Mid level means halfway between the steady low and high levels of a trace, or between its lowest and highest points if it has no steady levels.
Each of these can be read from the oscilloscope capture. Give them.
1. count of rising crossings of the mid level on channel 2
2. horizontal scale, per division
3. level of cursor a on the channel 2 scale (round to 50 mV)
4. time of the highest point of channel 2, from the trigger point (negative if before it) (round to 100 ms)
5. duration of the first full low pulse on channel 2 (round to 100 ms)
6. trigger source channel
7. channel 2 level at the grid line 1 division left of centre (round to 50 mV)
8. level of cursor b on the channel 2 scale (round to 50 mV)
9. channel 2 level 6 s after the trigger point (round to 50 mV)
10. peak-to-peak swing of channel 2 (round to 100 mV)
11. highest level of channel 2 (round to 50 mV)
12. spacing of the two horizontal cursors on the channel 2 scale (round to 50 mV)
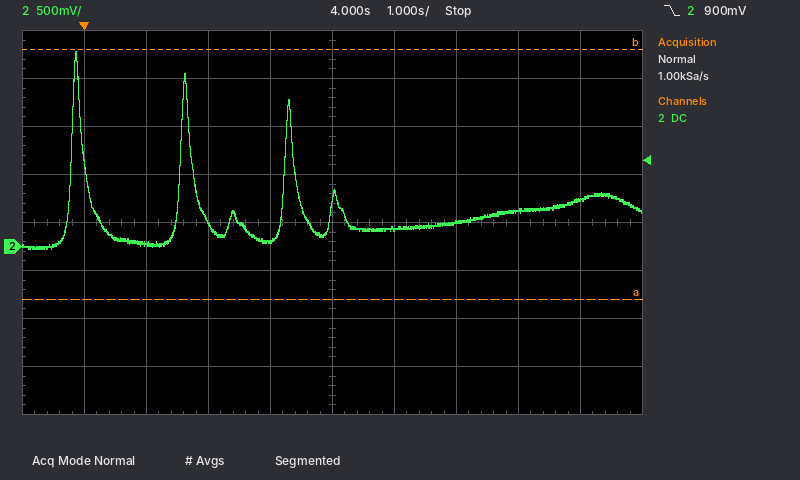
3
1 s
-550 mV
-100 ms
1.6 s
channel 2
50 mV
2.05 V
250 mV
2.10 V
2.05 V
2.60 V
